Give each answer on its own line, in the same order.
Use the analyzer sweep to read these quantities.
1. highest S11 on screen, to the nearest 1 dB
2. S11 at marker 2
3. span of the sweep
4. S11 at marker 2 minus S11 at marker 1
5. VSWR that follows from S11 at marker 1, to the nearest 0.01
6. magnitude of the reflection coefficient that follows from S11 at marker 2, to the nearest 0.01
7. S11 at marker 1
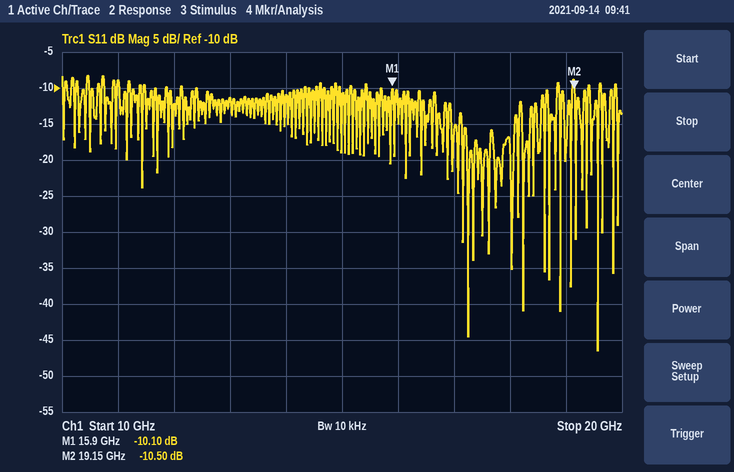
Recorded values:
-8 dB
-10.50 dB
10 GHz
-0.40 dB
1.91
0.30
-10.10 dB
